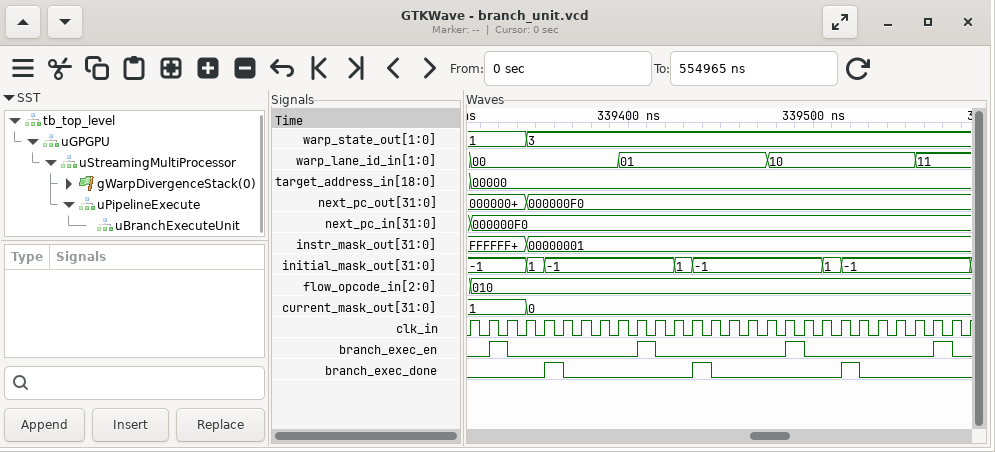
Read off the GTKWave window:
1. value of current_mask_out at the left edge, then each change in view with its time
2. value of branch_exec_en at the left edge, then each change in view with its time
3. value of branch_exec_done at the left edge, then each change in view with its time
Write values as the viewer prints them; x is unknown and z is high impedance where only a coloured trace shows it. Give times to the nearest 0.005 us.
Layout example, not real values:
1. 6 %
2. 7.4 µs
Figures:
1. 1, 0 at 339.345 us
2. 0, 1 at 339.325 us, 0 at 339.335 us, 1 at 339.405 us, 0 at 339.415 us, 1 at 339.485 us, 0 at 339.495 us, 1 at 339.565 us, 0 at 339.575 us
3. 0, 1 at 339.355 us, 0 at 339.365 us, 1 at 339.435 us, 0 at 339.445 us, 1 at 339.515 us, 0 at 339.525 us
